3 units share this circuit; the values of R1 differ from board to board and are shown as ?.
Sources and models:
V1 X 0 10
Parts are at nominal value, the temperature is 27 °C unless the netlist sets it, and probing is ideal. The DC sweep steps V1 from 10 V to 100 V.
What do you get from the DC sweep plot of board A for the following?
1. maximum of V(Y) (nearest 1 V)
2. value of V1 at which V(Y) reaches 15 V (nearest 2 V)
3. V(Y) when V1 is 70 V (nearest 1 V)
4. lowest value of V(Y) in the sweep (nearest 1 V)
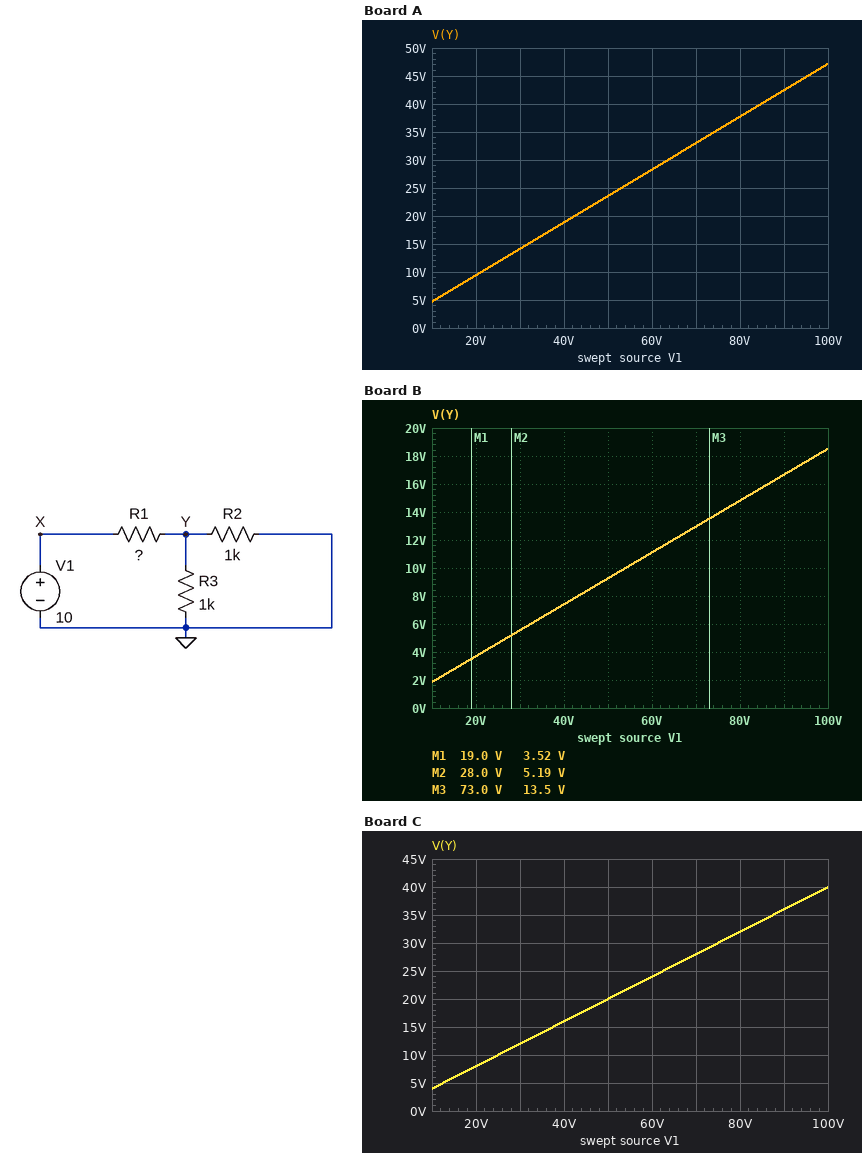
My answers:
47 V
32 V
33 V
5 V
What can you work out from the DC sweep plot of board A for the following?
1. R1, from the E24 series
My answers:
560 Ω
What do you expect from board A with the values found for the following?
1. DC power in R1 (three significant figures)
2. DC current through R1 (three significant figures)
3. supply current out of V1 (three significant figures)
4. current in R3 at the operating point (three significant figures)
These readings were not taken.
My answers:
49.8 mW
9.43 mA
9.43 mA
4.72 mA
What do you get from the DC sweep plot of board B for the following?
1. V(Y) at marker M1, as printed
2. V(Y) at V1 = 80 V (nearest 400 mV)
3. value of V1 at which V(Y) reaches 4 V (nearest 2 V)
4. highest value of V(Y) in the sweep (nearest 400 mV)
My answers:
3.52 V
14.8 V
22 V
18.4 V
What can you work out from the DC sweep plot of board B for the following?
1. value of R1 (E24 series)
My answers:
2.2 kΩ
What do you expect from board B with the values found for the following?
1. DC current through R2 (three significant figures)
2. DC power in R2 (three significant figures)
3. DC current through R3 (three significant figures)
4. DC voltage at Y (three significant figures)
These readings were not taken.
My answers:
1.85 mA
3.43 mW
1.85 mA
1.85 V
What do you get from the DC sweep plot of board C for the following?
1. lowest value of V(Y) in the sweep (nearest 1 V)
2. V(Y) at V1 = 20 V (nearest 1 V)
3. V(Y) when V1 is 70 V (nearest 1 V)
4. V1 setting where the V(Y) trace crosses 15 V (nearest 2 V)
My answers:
4 V
8 V
28 V
38 V
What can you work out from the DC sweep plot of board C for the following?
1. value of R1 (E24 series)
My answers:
750 Ω
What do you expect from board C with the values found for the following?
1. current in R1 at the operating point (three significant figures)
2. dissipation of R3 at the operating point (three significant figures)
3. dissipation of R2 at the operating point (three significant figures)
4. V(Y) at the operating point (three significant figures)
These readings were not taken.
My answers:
8.00 mA
16.0 mW
16.0 mW
4.00 V
